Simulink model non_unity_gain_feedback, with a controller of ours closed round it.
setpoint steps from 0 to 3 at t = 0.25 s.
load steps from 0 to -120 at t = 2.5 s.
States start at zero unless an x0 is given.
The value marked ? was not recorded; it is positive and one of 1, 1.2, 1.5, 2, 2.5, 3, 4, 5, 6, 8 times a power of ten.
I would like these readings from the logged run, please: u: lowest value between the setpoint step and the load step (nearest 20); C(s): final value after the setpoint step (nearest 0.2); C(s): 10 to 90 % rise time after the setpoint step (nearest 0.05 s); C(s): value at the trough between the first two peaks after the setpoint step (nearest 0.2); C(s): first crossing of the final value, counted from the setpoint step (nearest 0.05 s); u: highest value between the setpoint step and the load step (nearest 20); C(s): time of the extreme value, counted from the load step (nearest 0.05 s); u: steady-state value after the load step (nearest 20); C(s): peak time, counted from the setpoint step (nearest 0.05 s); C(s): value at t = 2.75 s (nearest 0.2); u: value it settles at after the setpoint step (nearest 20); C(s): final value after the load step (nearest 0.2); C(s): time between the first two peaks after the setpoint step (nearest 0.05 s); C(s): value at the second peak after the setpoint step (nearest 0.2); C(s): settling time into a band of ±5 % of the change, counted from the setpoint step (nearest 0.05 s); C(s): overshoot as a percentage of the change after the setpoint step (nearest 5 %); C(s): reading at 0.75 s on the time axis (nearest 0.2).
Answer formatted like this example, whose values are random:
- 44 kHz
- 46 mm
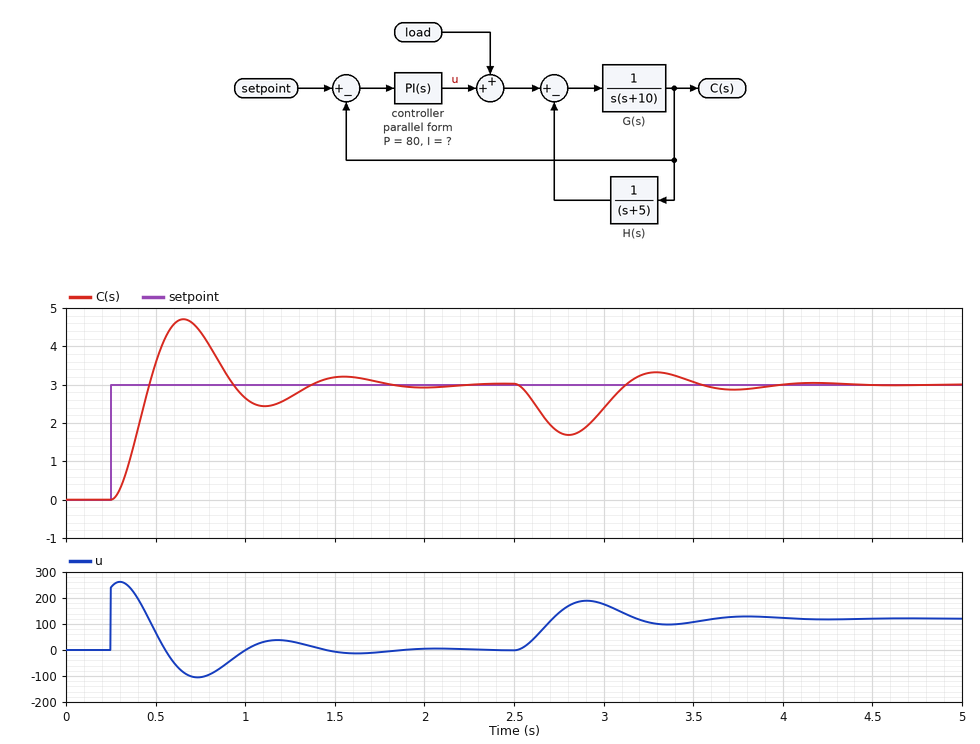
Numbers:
- -100
- 3.0
- 0.15 s
- 2.4
- 0.20 s
- 260
- 0.30 s
- 120
- 0.40 s
- 1.8
- 0
- 3.0
- 0.90 s
- 3.2
- 1.40 s
- 55 %
- 4.4
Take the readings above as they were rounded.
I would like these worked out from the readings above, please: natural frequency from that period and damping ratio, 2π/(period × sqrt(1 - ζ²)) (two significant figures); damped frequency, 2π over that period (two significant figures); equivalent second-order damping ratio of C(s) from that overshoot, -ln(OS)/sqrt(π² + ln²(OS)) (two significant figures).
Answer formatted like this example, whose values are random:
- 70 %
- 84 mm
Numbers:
- 7.1 rad/s
- 7.0 rad/s
- 0.19
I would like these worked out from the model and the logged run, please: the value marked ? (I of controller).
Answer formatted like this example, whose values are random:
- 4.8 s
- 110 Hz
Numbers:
- 300
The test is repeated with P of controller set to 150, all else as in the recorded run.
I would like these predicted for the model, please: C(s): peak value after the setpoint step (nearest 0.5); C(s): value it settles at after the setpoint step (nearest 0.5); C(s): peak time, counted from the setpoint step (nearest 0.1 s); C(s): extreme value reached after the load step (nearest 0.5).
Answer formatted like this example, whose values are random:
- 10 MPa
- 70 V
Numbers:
- 4.5
- 3.0
- 0.3 s
- 2.0
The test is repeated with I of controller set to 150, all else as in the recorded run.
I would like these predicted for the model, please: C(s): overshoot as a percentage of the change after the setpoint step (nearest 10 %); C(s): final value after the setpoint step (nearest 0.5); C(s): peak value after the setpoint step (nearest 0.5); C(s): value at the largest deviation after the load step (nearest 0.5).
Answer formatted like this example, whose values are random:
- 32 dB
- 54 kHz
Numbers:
- 40 %
- 3.0
- 4.0
- 1.5
